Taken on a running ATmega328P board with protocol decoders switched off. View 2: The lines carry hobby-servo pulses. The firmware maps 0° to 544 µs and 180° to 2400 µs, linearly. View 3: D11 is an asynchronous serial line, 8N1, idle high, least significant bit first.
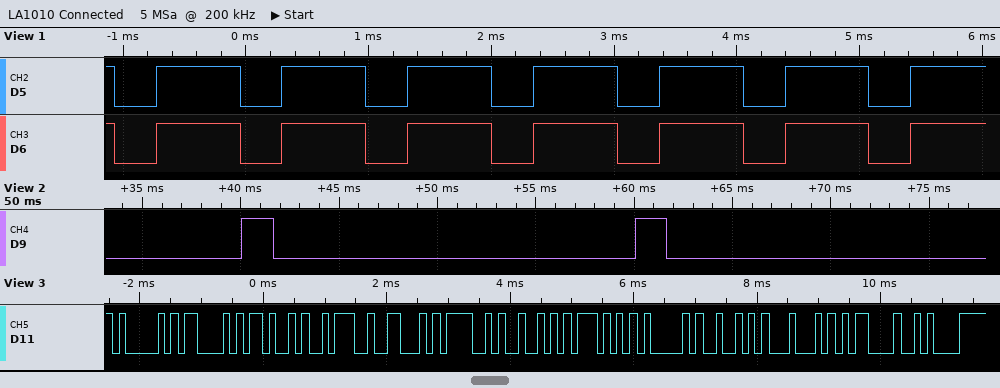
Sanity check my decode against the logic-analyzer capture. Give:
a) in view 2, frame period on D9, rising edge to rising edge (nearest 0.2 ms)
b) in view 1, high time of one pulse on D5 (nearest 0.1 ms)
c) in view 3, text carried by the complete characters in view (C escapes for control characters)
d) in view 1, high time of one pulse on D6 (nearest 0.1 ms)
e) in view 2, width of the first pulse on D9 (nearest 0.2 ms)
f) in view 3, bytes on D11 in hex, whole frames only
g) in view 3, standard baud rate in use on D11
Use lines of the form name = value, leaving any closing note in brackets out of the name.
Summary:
in view 2, frame period on D9, rising edge to rising edge = 20.0 ms
in view 1, high time of one pulse on D5 = 0.7 ms
in view 3, text carried by the complete characters in view = "ACK:FORWARD\r\n"
in view 1, high time of one pulse on D6 = 0.7 ms
in view 2, width of the first pulse on D9 = 1.6 ms
in view 3, bytes on D11 in hex, whole frames only = 0x41 0x43 0x4B 0x3A 0x46 0x4F 0x52 0x57 0x41 0x52 0x44 0x0D 0x0A
in view 3, standard baud rate in use on D11 = 9600 baud
